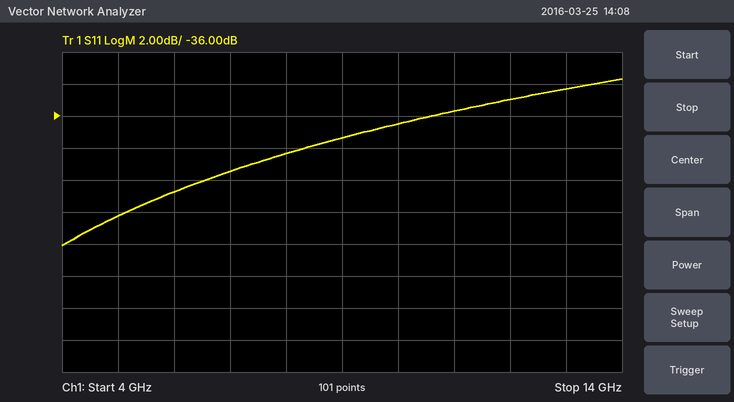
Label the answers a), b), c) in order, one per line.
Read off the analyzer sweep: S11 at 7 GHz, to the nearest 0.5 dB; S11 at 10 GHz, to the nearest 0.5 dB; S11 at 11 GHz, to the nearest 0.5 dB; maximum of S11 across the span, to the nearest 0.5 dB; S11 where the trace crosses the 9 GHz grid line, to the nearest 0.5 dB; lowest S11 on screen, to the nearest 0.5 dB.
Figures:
a) -39.5 dB
b) -36.5 dB
c) -35.5 dB
d) -33.5 dB
e) -37.5 dB
f) -44.0 dB
